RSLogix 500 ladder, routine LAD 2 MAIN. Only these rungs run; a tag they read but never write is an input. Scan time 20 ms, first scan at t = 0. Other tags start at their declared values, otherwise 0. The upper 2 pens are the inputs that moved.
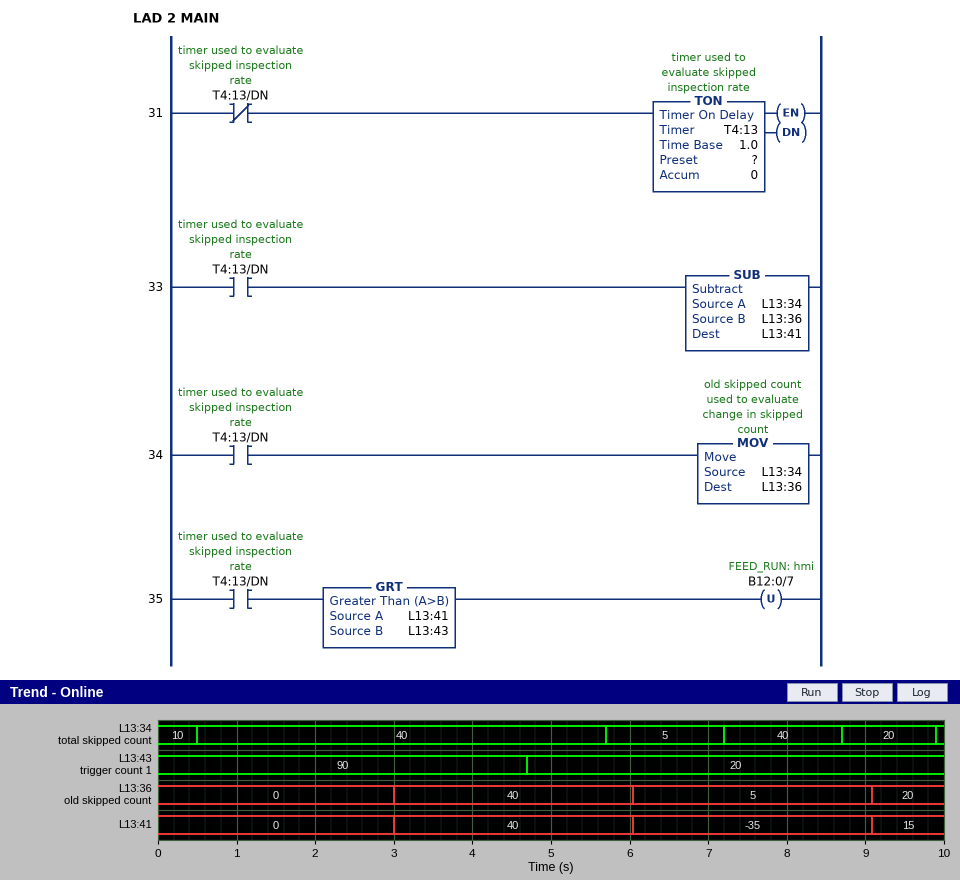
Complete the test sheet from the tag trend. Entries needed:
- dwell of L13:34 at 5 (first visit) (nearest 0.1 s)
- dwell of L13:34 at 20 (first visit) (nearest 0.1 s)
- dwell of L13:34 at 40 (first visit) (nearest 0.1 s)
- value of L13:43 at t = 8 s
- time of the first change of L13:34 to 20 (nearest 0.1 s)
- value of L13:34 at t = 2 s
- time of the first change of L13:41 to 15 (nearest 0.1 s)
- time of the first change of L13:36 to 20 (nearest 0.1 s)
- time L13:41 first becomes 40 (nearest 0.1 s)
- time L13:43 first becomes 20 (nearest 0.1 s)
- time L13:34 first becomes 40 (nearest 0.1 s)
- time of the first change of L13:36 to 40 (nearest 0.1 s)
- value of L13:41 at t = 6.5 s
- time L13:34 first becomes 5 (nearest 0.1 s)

1.5 s
1.2 s
5.2 s
20
8.7 s
40
9.1 s
9.1 s
3.0 s
4.7 s
0.5 s
3.0 s
-35
5.7 s
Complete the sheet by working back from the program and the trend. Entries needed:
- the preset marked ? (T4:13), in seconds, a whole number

3 s
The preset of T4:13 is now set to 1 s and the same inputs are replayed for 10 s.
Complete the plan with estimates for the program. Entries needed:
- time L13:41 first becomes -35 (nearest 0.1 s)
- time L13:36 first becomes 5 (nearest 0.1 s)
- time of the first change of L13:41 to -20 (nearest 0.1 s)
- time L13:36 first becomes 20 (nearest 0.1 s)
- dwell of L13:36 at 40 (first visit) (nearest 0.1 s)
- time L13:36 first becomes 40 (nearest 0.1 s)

6.2 s
6.2 s
9.3 s
9.3 s
5.2 s
1.0 s
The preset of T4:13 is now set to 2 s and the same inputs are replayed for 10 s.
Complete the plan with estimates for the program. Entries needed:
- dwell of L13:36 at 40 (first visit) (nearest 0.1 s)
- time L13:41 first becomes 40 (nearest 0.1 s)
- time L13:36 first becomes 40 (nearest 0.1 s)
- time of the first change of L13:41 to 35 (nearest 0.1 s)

4.1 s
2.0 s
2.0 s
8.1 s
